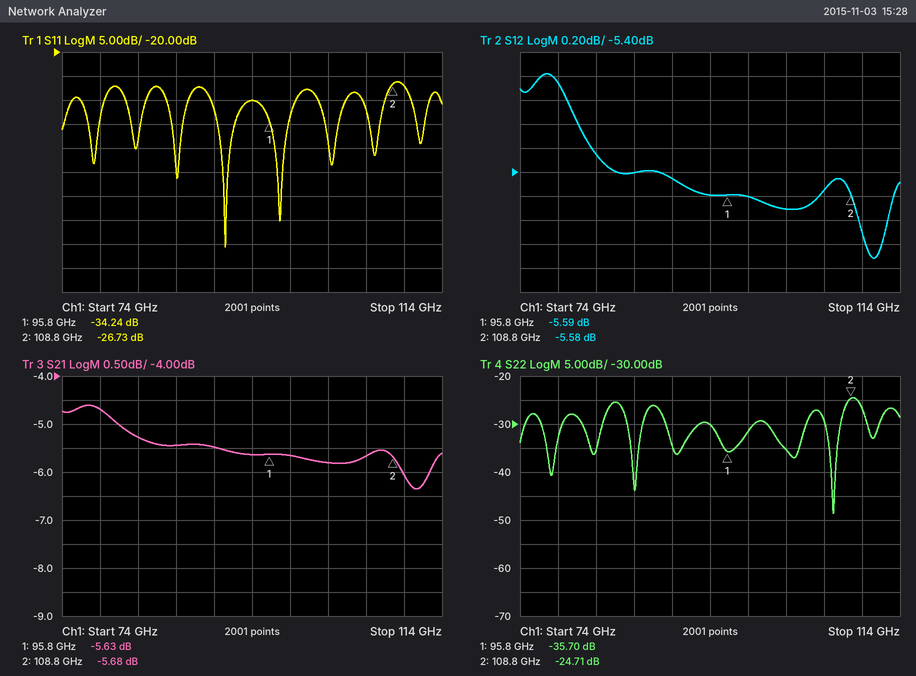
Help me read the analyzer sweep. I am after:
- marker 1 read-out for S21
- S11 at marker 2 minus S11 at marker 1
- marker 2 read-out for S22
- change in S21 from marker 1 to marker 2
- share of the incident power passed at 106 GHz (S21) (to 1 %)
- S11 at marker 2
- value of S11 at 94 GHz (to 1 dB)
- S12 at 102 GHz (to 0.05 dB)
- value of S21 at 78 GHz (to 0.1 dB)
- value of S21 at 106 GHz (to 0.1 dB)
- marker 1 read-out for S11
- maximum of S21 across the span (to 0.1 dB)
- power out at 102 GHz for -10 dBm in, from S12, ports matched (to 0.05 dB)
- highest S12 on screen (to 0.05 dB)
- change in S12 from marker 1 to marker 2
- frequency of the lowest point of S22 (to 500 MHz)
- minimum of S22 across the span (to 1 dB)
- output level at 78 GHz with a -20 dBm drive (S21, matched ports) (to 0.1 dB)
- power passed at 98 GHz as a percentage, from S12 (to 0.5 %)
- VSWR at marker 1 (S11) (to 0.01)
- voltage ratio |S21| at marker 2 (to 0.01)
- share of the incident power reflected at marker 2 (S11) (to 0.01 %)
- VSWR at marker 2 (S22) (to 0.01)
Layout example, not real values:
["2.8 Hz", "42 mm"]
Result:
["-5.63 dB", "7.51 dB", "-24.71 dB", "-0.05 dB", "27 %", "-26.73 dB", "-30 dB", "-5.70 dB", "-4.7 dB", "-5.7 dB", "-34.24 dB", "-4.6 dB", "-15.70 dBm", "-4.60 dB", "0.01 dB", "107.0 GHz", "-49 dB", "-24.7 dBm", "27.5 %", "1.04", "0.52", "0.21 %", "1.12"]
